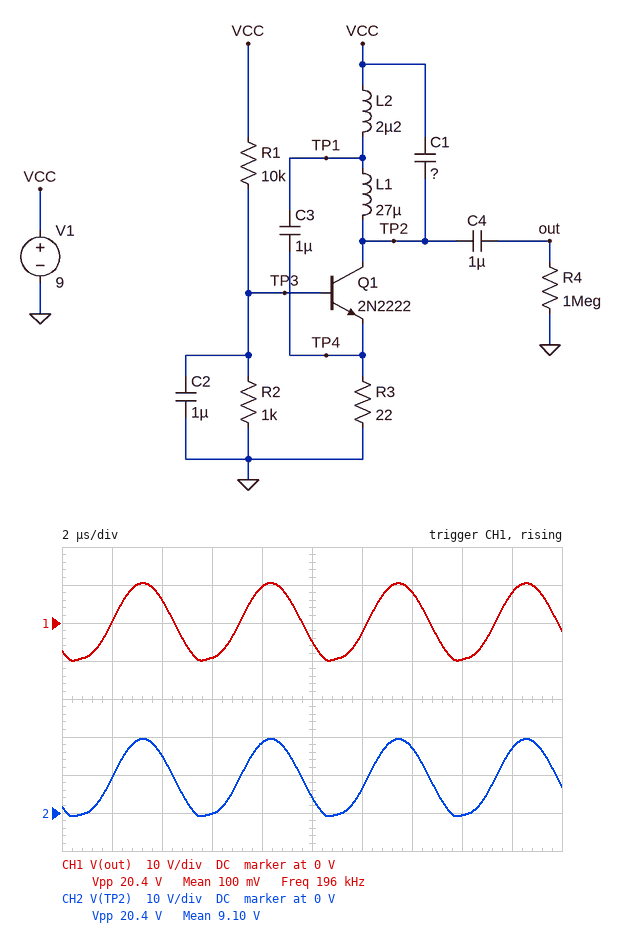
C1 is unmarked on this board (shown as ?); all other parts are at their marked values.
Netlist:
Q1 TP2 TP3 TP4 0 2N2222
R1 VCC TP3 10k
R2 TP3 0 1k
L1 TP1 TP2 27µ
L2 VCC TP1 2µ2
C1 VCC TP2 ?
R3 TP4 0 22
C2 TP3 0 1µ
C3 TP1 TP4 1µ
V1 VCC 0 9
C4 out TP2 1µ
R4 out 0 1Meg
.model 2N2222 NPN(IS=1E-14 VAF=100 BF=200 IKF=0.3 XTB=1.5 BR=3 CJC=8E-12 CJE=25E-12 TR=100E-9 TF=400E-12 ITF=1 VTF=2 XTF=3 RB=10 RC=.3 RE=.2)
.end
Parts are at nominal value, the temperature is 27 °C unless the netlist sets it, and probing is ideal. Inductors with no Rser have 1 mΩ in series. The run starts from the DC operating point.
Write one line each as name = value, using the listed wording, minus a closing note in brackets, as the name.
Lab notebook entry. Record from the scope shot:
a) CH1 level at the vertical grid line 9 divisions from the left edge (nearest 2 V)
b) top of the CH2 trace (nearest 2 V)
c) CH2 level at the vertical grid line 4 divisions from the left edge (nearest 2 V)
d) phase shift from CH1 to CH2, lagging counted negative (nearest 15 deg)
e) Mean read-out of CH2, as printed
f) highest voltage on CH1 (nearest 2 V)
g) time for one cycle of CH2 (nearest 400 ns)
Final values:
CH1 level at the vertical grid line 9 divisions from the left edge = 8 V
top of the CH2 trace = 20 V
CH2 level at the vertical grid line 4 divisions from the left edge = 18 V
phase shift from CH1 to CH2, lagging counted negative = 0 deg
Mean read-out of CH2, as printed = 9.10 V
highest voltage on CH1 = 10 V
time for one cycle of CH2 = 5.2 µs
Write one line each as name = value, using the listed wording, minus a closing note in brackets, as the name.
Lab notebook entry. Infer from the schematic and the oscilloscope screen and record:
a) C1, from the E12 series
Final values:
C1, from the E12 series = 22 nF
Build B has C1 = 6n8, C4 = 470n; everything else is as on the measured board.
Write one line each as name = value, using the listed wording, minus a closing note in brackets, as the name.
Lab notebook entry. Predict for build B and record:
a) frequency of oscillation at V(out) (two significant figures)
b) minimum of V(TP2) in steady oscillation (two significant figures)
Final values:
frequency of oscillation at V(out) = 350 kHz
minimum of V(TP2) in steady oscillation = -830 mV
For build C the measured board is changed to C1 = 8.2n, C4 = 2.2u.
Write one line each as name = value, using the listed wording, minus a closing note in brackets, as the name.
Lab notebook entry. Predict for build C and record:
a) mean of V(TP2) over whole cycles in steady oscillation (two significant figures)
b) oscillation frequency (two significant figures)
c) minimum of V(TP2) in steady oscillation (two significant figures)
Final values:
mean of V(TP2) over whole cycles in steady oscillation = 9.0 V
oscillation frequency = 320 kHz
minimum of V(TP2) in steady oscillation = -840 mV
